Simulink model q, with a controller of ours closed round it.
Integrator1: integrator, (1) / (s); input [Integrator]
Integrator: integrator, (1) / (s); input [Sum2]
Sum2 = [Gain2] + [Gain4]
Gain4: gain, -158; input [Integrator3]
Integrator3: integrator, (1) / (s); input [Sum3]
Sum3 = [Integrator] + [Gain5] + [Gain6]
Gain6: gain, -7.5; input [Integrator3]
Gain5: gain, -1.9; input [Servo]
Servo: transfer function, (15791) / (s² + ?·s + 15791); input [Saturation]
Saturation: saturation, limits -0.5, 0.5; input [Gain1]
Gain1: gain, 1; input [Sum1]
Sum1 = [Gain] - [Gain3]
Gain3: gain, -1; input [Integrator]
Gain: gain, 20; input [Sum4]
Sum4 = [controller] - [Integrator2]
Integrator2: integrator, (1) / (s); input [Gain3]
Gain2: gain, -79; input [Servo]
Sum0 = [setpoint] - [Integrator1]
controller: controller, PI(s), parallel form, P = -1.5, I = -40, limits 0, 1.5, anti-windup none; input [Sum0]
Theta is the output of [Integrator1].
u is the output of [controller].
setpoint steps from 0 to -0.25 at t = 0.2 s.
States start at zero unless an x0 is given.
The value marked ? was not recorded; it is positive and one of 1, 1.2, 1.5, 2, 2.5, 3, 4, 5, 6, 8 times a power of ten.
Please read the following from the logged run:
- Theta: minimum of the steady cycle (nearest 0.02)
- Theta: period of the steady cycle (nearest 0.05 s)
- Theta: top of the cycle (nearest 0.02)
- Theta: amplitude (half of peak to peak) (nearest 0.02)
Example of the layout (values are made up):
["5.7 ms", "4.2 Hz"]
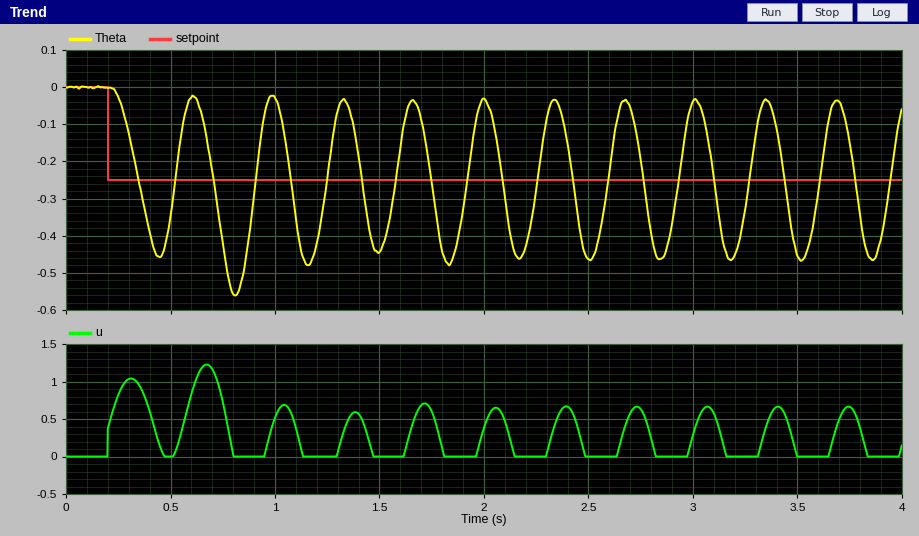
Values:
["-0.46", "0.35 s", "-0.04", "0.22"]
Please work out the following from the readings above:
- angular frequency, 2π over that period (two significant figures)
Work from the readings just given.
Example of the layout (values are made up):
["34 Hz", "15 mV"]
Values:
["18 rad/s"]
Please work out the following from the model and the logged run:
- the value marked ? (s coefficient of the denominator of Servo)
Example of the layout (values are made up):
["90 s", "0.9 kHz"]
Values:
["200"]
